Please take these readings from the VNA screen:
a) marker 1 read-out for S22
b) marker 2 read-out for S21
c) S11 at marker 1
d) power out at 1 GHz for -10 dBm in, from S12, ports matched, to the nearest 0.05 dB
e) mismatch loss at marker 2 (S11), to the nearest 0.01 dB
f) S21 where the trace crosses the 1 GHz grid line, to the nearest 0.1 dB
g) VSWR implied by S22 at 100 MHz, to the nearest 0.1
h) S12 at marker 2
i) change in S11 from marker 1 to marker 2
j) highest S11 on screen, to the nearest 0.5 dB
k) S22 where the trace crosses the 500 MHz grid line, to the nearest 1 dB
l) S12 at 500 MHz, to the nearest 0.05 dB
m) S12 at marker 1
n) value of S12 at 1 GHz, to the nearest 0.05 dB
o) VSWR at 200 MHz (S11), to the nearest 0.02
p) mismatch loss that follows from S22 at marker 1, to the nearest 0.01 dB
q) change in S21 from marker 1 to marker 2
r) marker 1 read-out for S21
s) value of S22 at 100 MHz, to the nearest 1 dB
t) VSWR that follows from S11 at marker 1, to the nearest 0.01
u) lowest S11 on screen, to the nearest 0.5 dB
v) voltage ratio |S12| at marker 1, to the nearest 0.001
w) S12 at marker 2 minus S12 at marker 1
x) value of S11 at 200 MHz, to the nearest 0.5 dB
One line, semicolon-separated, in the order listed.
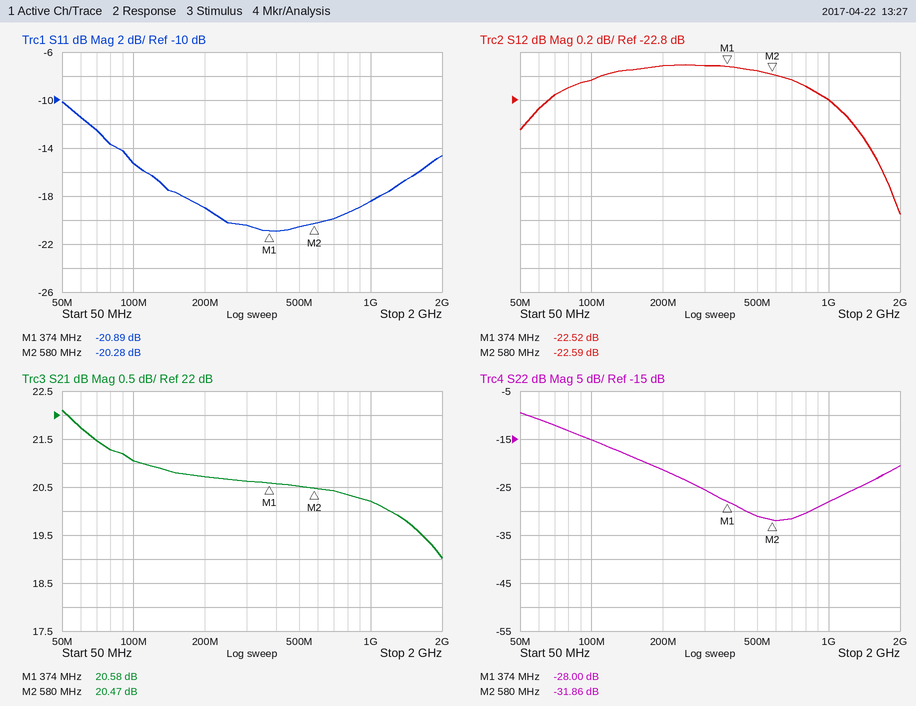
-28.00 dB; 20.47 dB; -20.89 dB; -32.80 dBm; 0.04 dB; 20.2 dB; 1.4; -22.59 dB; 0.61 dB; -10.0 dB; -31 dB; -22.55 dB; -22.52 dB; -22.80 dB; 1.26; 0.01 dB; -0.11 dB; 20.58 dB; -15 dB; 1.20; -21.0 dB; 0.075; -0.07 dB; -19.0 dB
